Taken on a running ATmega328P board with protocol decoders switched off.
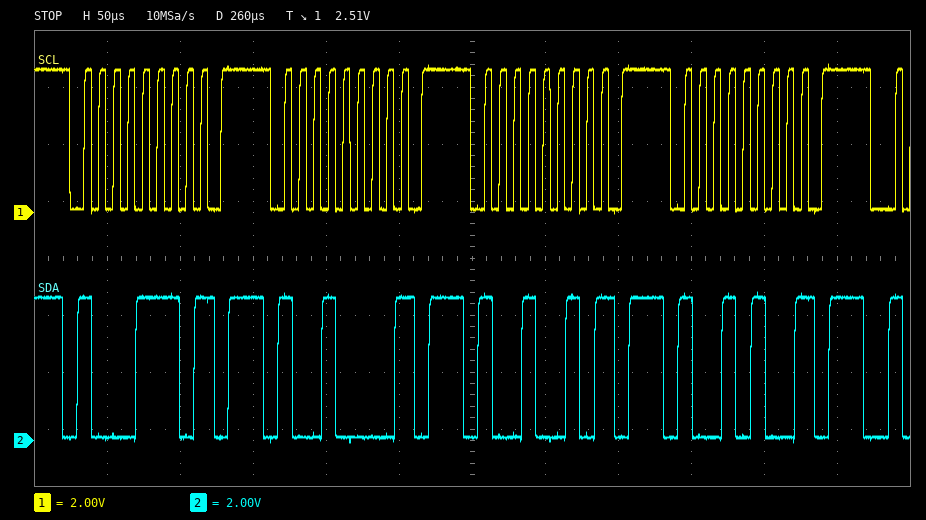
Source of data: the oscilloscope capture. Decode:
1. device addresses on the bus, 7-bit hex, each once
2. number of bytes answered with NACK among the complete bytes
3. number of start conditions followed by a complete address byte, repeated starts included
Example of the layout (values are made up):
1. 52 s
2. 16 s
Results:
1. 0x47 0x48 0x49 0x4A
2. 4
3. 4
